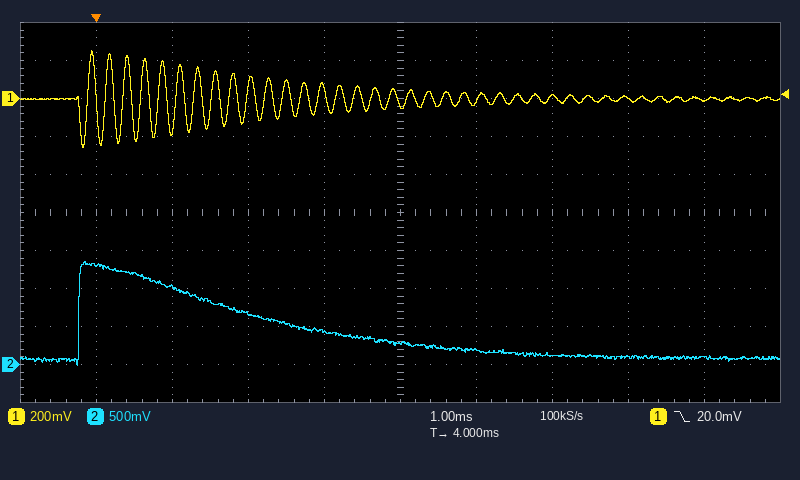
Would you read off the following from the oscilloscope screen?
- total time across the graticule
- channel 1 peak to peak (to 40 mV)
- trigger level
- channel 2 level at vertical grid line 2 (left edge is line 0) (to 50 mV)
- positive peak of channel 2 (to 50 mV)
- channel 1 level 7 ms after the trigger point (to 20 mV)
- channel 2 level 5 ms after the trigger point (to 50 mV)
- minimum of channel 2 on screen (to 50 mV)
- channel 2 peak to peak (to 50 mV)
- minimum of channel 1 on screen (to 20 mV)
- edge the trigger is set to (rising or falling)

10 ms
520 mV
20.0 mV
1.00 V
1.35 V
0 mV
200 mV
0 mV
1.35 V
-260 mV
falling
